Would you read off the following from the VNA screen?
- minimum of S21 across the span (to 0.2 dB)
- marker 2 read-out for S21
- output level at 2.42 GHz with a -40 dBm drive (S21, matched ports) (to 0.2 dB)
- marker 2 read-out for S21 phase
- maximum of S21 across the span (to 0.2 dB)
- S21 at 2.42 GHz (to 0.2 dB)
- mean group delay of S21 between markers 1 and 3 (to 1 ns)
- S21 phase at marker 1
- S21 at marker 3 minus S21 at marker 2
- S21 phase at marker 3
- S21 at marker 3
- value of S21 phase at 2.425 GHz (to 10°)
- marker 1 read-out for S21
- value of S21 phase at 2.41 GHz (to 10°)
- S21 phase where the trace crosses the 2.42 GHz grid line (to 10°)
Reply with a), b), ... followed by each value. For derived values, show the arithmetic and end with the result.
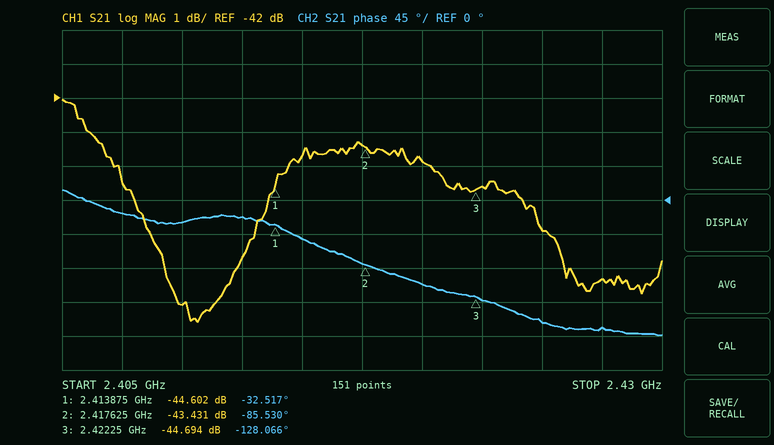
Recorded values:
a) -48.6 dB
b) -43.431 dB
c) -40 dBm + (-43.8 dB) = -83.8 dBm
d) -85.530°
e) -42.0 dB
f) -43.8 dB
g) −(-128.066° − (-32.517°))/(360° × 8.375 MHz) ≈ 32 ns
h) -32.517°
i) -44.694 − (-43.431) = -1.263 dB
j) -128.066°
k) -44.694 dB
l) -160°
m) -44.602 dB
n) -30°
o) -110°
